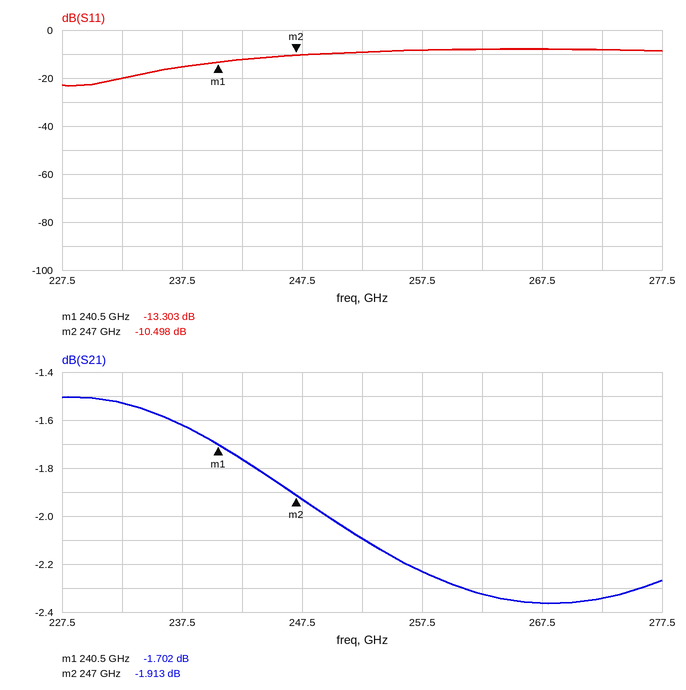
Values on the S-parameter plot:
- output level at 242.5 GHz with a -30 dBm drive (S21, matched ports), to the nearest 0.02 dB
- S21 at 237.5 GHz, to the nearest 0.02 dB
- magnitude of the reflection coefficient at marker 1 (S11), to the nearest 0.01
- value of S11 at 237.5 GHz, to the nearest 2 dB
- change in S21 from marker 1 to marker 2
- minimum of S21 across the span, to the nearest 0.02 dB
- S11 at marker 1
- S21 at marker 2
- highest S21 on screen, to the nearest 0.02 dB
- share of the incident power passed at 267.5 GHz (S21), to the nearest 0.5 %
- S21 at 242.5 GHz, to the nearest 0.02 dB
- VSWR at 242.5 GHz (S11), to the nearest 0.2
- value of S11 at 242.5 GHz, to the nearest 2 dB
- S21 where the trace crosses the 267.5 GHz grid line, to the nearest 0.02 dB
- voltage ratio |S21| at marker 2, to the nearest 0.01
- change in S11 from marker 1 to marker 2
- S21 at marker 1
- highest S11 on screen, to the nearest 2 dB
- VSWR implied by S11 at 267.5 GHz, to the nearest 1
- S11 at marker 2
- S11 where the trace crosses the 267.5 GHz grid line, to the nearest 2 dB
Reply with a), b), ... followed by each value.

a) -31.76 dBm
b) -1.62 dB
c) 0.22
d) -16 dB
e) -0.211 dB
f) -2.36 dB
g) -13.303 dB
h) -1.913 dB
i) -1.50 dB
j) 58.0 %
k) -1.76 dB
l) 1.6
m) -12 dB
n) -2.36 dB
o) 0.80
p) 2.805 dB
q) -1.702 dB
r) -8 dB
s) 2
t) -10.498 dB
u) -8 dB
